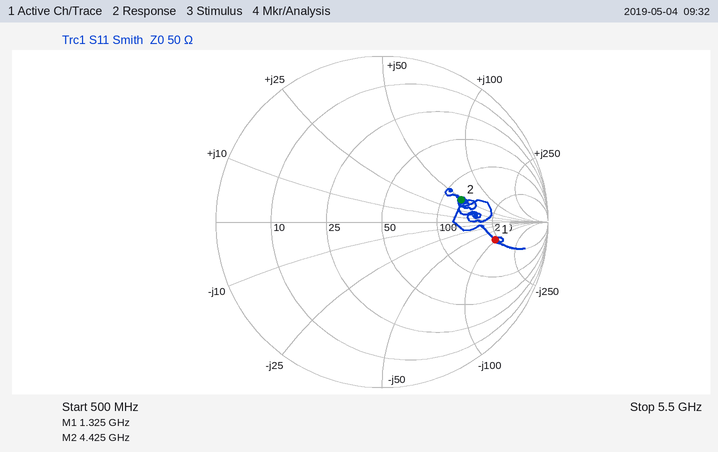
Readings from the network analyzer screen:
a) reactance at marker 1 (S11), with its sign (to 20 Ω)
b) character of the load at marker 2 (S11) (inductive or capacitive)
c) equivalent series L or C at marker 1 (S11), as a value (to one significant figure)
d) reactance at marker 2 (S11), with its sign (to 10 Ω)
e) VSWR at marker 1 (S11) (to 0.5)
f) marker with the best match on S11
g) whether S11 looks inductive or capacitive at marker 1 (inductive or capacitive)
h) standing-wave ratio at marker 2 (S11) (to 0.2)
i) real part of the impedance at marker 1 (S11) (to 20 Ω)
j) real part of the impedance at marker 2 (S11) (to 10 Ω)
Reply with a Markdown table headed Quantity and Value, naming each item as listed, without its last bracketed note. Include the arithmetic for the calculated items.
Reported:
| Quantity | Value |
|---|---|
| reactance at marker 1 (S11), with its sign | -100 Ω |
| character of the load at marker 2 (S11) | inductive |
| equivalent series L or C at marker 1 (S11), as a value | C = 1/(2π × 1.325 GHz × 100 Ω) ≈ 1 pF |
| reactance at marker 2 (S11), with its sign | +50 Ω |
| VSWR at marker 1 (S11) | 5.5 |
| marker with the best match on S11 | marker 2 |
| whether S11 looks inductive or capacitive at marker 1 | capacitive |
| standing-wave ratio at marker 2 (S11) | 3.0 |
| real part of the impedance at marker 1 (S11) | 240 Ω |
| real part of the impedance at marker 2 (S11) | 130 Ω |
